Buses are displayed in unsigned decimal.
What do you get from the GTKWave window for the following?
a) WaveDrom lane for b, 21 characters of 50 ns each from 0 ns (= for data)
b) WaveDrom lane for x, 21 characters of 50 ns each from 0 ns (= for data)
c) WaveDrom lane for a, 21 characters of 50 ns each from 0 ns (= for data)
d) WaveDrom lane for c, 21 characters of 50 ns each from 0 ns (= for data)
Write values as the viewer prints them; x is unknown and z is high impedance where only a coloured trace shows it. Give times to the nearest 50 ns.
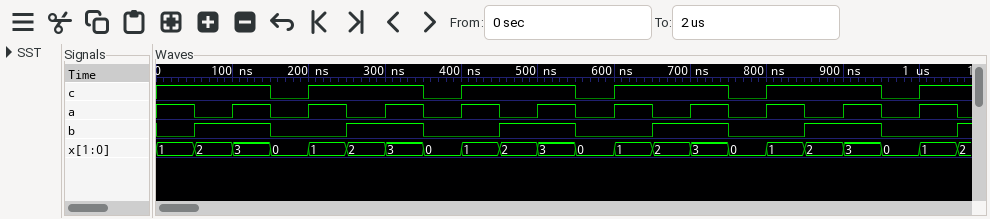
{name: 'b', wave: '01.0.1.0.1.0.1.0.1.0.'}
{name: 'x', wave: '=====================', data: '1 2 3 0 1 2 3 0 1 2 3 0 1 2 3 0 1 2 3 0 1'}
{name: 'a', wave: '101010101010101010101'}
{name: 'c', wave: '1..01..01..01..01..01'}
